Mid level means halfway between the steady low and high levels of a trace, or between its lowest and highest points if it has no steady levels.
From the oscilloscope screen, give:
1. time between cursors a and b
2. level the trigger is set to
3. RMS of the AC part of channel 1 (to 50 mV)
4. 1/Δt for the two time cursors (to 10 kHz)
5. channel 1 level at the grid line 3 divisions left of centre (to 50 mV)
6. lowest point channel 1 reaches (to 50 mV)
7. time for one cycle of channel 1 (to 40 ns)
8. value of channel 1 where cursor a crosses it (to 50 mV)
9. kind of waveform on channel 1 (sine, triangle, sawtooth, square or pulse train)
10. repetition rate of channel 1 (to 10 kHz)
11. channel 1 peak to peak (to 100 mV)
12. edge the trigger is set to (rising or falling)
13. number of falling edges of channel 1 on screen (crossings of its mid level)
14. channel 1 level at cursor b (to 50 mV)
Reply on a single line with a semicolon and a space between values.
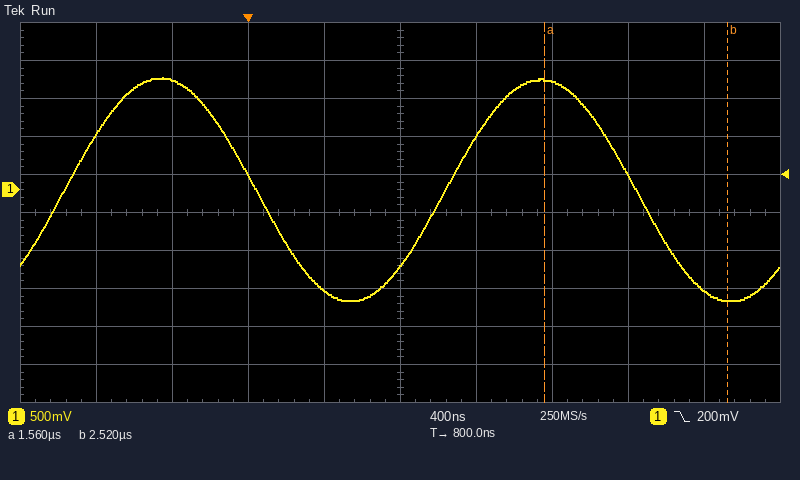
960 ns; 200 mV; 1.05 V; 1.04 MHz; 1.45 V; -1.45 V; 2.00 µs; 1.45 V; sine; 500 kHz; 2.90 V; falling; 2; -1.45 V
